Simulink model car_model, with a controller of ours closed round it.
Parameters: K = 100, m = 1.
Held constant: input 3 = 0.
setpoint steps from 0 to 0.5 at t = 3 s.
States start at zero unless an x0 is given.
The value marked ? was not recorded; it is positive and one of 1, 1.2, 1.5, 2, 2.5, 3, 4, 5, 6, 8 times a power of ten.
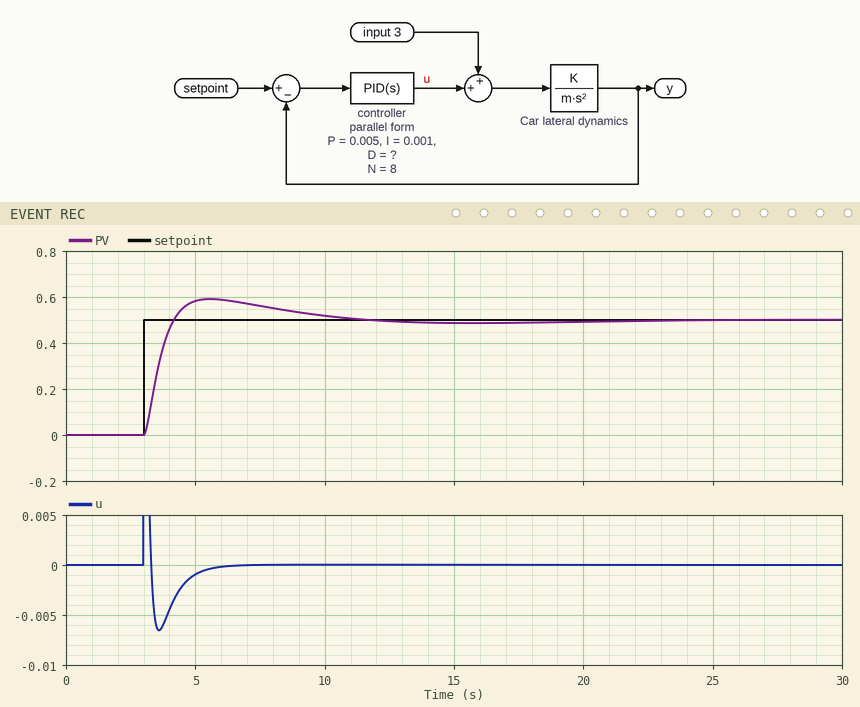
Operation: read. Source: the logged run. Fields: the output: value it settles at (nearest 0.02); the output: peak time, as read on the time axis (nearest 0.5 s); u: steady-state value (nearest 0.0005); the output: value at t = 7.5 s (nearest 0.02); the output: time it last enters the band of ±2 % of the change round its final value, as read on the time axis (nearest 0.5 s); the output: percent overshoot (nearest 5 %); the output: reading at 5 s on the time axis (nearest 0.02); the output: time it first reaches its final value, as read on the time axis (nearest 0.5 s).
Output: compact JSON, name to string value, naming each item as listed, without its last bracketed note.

{"the output: value it settles at": "0.50", "the output: peak time, as read on the time axis": "5.5 s", "u: steady-state value": "0.0000", "the output: value at t = 7.5 s": "0.56", "the output: time it last enters the band of ±2 % of the change round its final value, as read on the time axis": "19.0 s", "the output: percent overshoot": "20 %", "the output: reading at 5 s on the time axis": "0.58", "the output: time it first reaches its final value, as read on the time axis": "4.0 s"}
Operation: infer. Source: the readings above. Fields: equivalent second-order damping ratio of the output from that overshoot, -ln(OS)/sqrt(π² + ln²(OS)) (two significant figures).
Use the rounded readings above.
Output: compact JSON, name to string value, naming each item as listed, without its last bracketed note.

{"equivalent second-order damping ratio of the output from that overshoot, -ln(OS)/sqrt(π² + ln²(OS))": "0.46"}
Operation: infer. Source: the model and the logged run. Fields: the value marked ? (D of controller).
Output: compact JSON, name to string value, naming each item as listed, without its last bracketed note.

{"the value marked ?": "0.015"}
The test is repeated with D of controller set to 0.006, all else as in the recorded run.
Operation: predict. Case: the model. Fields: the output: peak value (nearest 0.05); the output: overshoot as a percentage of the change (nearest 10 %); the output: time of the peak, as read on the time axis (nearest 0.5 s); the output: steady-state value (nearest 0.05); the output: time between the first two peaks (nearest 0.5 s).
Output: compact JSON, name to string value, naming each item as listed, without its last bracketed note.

{"the output: peak value": "0.75", "the output: overshoot as a percentage of the change": "50 %", "the output: time of the peak, as read on the time axis": "6.5 s", "the output: steady-state value": "0.50", "the output: time between the first two peaks": "10.0 s"}
